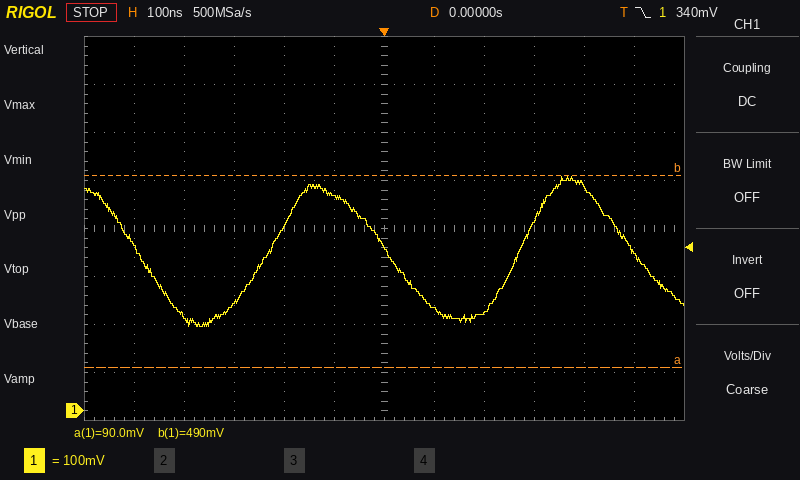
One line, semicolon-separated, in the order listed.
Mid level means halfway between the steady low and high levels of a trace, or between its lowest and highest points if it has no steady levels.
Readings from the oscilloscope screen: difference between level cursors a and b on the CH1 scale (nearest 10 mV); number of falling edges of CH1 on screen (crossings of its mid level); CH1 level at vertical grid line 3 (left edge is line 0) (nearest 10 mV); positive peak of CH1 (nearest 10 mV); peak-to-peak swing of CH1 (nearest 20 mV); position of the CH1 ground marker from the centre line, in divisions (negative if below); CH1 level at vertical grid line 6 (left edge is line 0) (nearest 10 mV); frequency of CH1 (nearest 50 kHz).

400 mV; 3; 220 mV; 490 mV; 320 mV; -3.8 div; 340 mV; 2.00 MHz
